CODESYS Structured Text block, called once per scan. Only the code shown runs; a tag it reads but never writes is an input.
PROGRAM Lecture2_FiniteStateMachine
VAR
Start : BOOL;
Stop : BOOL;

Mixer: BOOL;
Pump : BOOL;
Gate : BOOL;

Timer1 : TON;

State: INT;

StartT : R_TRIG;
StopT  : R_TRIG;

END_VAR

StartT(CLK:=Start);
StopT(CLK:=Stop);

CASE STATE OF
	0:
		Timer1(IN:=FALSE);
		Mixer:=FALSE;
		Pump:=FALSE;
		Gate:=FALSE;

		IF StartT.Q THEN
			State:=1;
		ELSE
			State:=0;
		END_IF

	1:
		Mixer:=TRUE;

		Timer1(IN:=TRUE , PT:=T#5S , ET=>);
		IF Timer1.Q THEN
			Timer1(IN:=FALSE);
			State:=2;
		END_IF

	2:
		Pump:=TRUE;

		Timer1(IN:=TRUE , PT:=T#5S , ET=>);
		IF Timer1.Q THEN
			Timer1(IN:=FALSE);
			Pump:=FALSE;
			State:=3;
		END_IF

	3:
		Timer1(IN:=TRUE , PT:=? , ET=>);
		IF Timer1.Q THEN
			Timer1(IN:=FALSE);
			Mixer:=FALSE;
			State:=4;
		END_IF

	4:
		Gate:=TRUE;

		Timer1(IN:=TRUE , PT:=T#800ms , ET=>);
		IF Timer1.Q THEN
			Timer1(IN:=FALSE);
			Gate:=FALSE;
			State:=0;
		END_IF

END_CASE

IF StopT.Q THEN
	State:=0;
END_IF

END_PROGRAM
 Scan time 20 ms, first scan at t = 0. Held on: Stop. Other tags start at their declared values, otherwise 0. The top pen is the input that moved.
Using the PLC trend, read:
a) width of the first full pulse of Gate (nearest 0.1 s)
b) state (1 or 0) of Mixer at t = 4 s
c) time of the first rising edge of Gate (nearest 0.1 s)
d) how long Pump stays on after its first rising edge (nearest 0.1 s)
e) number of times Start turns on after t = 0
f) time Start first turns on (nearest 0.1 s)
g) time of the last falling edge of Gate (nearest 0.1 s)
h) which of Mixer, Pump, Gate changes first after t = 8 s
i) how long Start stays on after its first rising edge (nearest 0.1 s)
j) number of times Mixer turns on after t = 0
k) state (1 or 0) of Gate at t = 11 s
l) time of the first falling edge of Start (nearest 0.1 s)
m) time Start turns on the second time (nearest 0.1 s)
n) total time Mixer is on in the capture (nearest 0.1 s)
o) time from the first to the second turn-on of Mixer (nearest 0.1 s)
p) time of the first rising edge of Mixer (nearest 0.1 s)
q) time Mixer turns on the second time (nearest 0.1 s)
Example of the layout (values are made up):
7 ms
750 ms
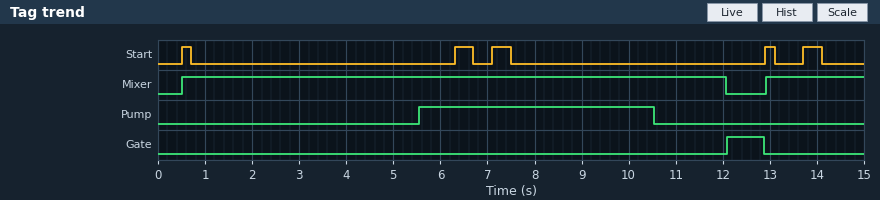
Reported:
0.8 s
1
12.1 s
5.0 s
5
0.5 s
12.9 s
Pump
0.2 s
2
0
0.7 s
6.3 s
13.6 s
12.4 s
0.5 s
12.9 s
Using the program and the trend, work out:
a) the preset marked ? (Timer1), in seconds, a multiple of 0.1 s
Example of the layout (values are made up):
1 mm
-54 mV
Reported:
1.5 s
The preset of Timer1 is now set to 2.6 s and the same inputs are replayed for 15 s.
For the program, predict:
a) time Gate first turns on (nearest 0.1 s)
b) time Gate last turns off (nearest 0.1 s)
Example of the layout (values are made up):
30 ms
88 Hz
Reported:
13.2 s
14.0 s
